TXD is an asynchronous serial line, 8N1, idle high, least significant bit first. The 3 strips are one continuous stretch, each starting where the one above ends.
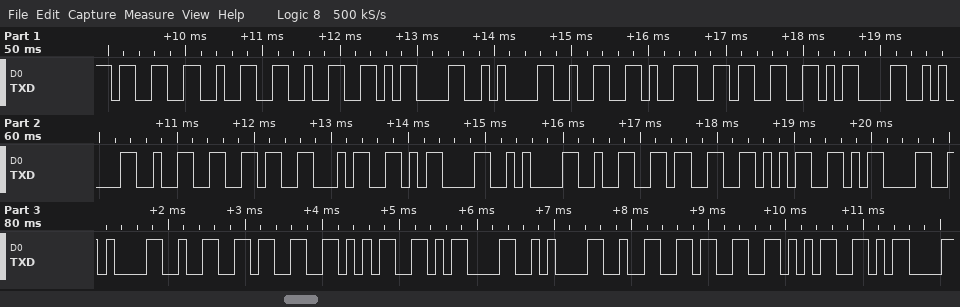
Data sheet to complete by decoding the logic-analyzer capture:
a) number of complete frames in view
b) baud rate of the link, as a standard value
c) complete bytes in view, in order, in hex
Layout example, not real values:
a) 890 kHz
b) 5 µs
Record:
a) 29
b) 9600 baud
c) 33 32 32 0D 0A 32 39 33 0D 0A 32 36 34 0D 0A 32 33 35 0D 0A 32 33 35 0D 0A 32 33 35 0D
